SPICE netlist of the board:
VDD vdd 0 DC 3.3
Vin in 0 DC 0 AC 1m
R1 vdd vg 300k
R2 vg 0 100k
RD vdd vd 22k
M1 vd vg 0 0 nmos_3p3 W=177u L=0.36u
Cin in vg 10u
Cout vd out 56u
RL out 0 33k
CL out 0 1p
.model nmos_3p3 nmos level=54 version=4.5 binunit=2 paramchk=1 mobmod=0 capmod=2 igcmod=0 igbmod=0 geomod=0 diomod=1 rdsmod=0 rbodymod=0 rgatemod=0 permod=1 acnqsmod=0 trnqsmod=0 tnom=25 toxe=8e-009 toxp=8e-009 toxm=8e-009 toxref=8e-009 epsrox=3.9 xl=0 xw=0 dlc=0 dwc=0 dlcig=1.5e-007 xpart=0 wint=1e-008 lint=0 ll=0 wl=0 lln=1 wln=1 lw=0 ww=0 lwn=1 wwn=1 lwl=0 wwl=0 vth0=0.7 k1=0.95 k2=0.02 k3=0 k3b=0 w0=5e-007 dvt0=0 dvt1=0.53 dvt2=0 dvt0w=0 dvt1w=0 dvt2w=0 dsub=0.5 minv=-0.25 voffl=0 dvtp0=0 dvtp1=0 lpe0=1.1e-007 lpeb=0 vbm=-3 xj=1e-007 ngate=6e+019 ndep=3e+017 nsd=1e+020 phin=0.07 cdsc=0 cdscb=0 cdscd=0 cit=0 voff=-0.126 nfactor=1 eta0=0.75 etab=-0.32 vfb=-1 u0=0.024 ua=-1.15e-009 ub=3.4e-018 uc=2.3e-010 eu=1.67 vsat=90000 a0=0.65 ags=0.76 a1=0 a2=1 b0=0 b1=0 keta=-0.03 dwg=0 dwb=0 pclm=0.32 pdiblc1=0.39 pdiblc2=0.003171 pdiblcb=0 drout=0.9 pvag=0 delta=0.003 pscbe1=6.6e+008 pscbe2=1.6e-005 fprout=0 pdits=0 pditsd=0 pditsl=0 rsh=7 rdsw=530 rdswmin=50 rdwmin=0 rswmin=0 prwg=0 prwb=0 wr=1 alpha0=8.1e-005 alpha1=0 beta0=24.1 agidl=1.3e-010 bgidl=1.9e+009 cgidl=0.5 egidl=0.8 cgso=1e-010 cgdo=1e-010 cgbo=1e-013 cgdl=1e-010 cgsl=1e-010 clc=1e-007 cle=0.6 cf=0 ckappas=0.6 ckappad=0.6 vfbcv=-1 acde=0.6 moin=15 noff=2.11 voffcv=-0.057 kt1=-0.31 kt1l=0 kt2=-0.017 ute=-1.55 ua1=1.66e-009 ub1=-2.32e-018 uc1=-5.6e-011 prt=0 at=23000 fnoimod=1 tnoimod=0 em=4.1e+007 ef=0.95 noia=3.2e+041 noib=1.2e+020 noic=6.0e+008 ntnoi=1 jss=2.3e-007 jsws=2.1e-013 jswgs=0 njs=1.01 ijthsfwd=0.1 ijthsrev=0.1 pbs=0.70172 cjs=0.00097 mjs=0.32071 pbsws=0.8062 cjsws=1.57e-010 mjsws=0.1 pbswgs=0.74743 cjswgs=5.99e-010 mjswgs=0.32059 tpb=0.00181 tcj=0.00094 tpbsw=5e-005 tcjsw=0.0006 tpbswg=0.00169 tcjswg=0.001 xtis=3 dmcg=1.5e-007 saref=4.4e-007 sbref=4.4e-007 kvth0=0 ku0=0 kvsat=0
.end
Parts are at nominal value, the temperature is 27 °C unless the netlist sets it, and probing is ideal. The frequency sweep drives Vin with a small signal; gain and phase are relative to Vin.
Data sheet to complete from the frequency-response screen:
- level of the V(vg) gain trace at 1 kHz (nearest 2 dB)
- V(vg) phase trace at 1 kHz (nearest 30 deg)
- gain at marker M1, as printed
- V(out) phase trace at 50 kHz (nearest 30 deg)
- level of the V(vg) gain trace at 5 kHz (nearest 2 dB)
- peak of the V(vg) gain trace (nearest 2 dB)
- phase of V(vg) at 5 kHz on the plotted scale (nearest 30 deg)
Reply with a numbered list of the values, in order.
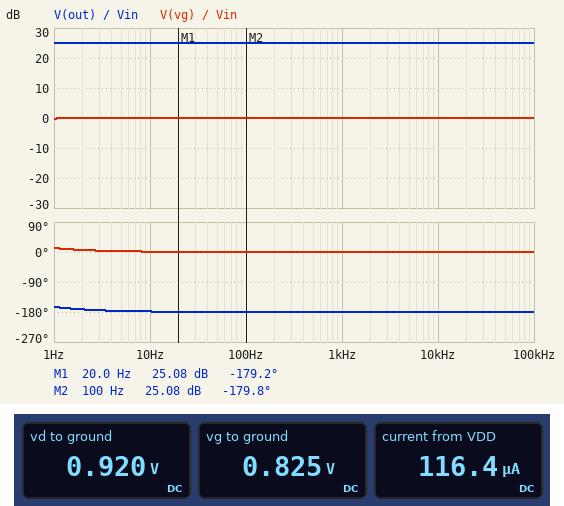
1. 0 dB
2. 0 deg
3. 25.08 dB
4. -180 deg
5. 0 dB
6. 0 dB
7. 0 deg
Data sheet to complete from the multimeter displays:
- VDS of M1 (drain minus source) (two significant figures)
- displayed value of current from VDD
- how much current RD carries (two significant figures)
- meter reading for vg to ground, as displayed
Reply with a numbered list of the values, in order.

1. 920 mV
2. 116.4 µA
3. 110 µA
4. 0.825 V
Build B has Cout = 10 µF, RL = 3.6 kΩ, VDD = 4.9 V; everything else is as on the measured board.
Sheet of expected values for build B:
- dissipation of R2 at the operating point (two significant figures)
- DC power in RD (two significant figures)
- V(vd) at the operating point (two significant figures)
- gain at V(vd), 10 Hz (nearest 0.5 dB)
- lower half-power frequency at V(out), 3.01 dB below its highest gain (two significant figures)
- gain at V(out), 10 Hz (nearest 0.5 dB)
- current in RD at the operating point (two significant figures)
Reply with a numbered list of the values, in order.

1. 15 µW
2. 1.1 mW
3. 12 mV
4. -31.0 dB
5. 4.4 Hz
6. -31.5 dB
7. 220 µA
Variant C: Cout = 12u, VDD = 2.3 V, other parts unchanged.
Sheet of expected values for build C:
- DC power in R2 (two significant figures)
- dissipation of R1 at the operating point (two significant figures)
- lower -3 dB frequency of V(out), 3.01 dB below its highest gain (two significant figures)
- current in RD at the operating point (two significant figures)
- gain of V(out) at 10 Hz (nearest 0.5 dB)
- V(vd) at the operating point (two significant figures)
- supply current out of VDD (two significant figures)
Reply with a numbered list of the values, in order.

1. 3.3 µW
2. 9.9 µW
3. 350 mHz
4. 620 nA
5. -13.5 dB
6. 2.3 V
7. 6.4 µA
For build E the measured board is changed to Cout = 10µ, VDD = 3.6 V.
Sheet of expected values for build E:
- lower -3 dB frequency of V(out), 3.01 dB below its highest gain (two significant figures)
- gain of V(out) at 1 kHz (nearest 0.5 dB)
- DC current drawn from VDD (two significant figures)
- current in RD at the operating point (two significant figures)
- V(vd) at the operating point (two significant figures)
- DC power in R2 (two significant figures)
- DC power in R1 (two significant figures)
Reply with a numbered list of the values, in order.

1. 550 mHz
2. -5.0 dB
3. 170 µA
4. 160 µA
5. 45 mV
6. 8.1 µW
7. 24 µW
